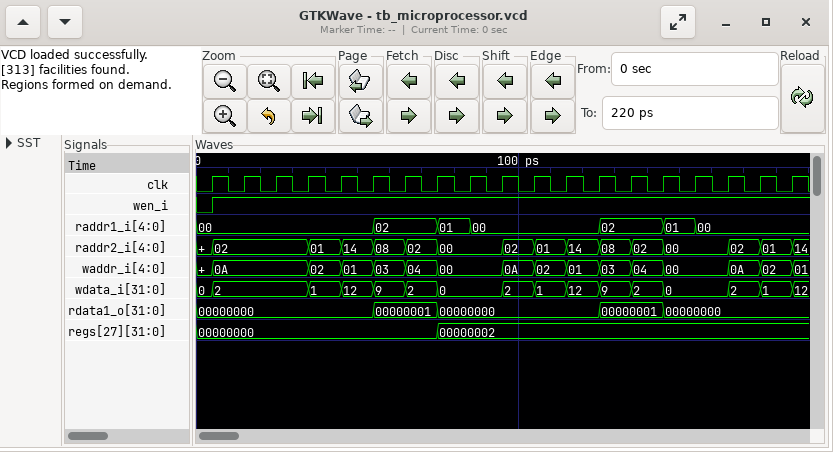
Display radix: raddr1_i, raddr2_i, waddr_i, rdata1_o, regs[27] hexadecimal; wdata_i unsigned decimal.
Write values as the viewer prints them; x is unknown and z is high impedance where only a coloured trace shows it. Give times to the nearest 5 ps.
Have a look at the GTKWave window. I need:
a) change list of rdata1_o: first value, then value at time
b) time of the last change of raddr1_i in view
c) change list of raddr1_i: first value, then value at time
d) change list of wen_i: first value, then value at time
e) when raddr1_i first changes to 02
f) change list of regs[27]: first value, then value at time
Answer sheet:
00000000, 00000001 at 55 ps, 00000000 at 75 ps, 00000001 at 125 ps, 00000000 at 145 ps
155 ps
00, 02 at 55 ps, 01 at 75 ps, 00 at 85 ps, 02 at 125 ps, 01 at 145 ps, 00 at 155 ps
0, 1 at 5 ps
55 ps
00000000, 00000002 at 75 ps
